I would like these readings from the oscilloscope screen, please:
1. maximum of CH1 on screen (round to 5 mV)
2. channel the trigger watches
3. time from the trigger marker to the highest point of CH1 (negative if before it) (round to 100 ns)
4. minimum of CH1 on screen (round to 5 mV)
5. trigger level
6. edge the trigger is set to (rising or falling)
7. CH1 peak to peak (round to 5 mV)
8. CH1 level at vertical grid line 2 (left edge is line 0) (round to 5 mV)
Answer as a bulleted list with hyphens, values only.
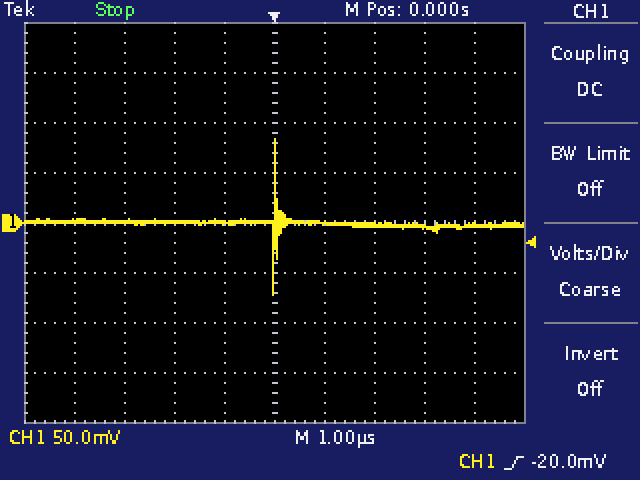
- 85 mV
- CH1
- 0.0 µs
- -70 mV
- -20.0 mV
- rising
- 155 mV
- 0 mV
